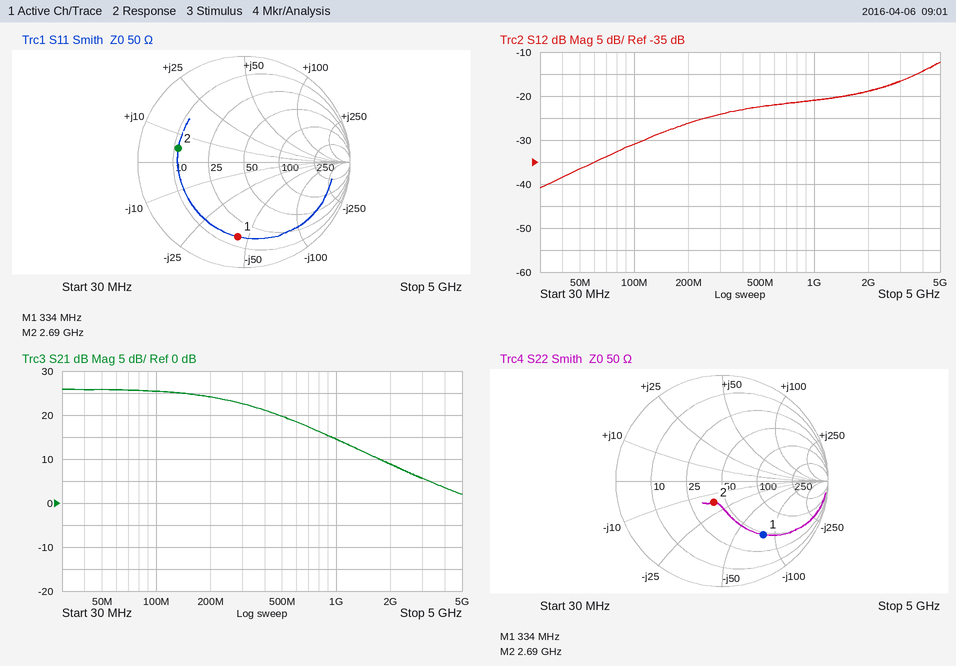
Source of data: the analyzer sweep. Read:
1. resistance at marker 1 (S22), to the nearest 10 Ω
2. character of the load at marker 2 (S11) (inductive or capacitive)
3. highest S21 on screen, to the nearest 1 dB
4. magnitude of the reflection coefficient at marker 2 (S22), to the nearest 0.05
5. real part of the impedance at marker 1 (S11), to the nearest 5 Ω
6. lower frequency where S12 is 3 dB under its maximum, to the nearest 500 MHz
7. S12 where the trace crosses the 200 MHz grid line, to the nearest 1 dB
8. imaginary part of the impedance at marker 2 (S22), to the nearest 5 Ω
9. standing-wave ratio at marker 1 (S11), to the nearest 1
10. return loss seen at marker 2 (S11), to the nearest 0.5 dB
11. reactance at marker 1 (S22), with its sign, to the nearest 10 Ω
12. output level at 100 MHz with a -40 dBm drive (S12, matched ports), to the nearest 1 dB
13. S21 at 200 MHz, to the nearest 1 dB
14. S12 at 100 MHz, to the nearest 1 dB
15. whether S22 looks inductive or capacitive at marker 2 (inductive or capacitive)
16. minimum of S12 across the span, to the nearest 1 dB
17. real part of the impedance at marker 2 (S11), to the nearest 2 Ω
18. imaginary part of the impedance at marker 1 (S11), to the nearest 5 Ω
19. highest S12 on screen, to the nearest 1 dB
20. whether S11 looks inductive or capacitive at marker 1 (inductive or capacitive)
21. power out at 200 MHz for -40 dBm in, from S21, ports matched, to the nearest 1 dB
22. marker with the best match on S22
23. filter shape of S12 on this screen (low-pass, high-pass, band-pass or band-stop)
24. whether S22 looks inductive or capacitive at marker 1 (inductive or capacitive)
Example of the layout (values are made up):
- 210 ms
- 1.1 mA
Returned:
- 50 Ω
- inductive
- 26 dB
- 0.20
- 15 Ω
- 3.5 GHz
- -26 dB
- -15 Ω
- 6
- 4.0 dB
- -80 Ω
- -71 dBm
- 24 dB
- -31 dB
- capacitive
- -41 dB
- 12 Ω
- -45 Ω
- -12 dB
- capacitive
- -16 dBm
- marker 2
- high-pass
- capacitive
